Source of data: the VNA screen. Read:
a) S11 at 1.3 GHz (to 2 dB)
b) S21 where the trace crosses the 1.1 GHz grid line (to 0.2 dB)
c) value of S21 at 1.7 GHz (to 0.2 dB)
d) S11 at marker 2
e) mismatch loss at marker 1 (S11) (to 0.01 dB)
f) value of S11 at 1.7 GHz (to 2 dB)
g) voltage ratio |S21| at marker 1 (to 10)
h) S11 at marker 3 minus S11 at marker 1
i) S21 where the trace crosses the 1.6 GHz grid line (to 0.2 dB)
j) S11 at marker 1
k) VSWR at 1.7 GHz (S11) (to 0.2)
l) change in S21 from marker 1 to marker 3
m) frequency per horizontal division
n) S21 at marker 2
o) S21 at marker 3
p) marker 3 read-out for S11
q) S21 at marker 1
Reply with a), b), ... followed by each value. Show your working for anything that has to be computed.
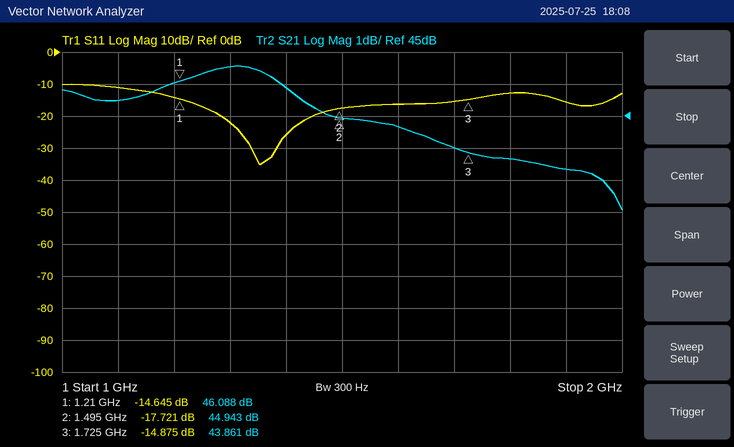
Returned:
a) -22 dB
b) 45.4 dB
c) 44.0 dB
d) -17.721 dB
e) −10 log10(1 − 10^(-14.645/10)) ≈ 0.15 dB
f) -16 dB
g) 10^(46.088/20) ≈ 202, so 200 to the nearest 10
h) -14.875 − (-14.645) = -0.230 dB
i) 44.6 dB
j) -14.645 dB
k) |Γ| = 10^(-16/20) = 0.1585; VSWR = (1 + 0.1585)/(1 − 0.1585) ≈ 1.4
l) 43.861 − (46.088) = -2.227 dB
m) 100 MHz
n) 44.943 dB
o) 43.861 dB
p) -14.875 dB
q) 46.088 dB
